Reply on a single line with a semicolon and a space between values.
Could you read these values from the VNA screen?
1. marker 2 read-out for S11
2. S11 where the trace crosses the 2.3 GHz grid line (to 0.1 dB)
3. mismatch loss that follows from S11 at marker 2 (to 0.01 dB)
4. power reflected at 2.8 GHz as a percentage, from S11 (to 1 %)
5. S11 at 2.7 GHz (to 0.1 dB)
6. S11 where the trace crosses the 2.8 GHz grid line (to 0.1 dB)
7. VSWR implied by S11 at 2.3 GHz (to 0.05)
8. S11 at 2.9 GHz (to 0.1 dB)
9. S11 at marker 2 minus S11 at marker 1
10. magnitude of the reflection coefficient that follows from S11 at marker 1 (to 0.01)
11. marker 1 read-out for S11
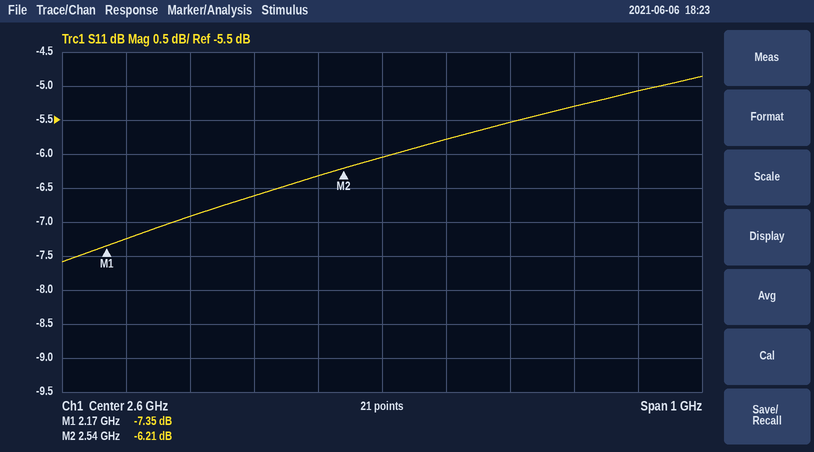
-6.21 dB; -6.9 dB; 1.19 dB; 28 %; -5.8 dB; -5.5 dB; 2.65; -5.3 dB; 1.14 dB; 0.43; -7.35 dB
